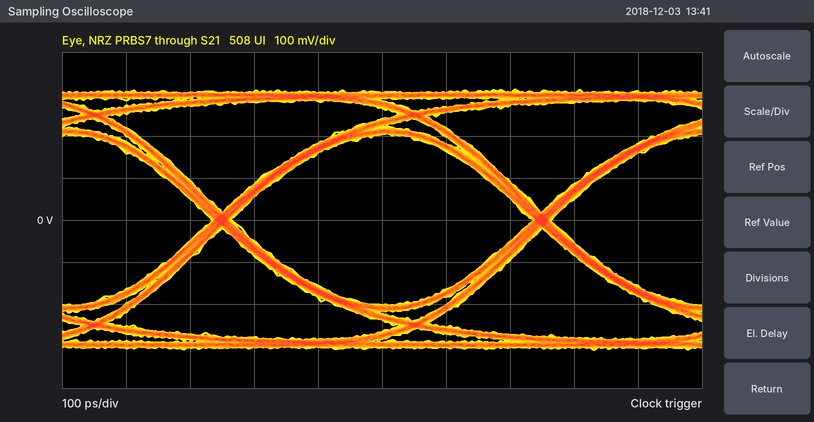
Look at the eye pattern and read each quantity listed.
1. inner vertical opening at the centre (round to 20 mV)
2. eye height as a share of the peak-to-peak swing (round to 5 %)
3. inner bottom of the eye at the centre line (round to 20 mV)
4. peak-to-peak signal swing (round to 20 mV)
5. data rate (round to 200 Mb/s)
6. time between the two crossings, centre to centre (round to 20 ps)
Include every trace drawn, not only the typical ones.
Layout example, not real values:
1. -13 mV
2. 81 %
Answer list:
1. 400 mV
2. 65 %
3. -200 mV
4. 620 mV
5. 2.0 Gb/s
6. 500 ps
